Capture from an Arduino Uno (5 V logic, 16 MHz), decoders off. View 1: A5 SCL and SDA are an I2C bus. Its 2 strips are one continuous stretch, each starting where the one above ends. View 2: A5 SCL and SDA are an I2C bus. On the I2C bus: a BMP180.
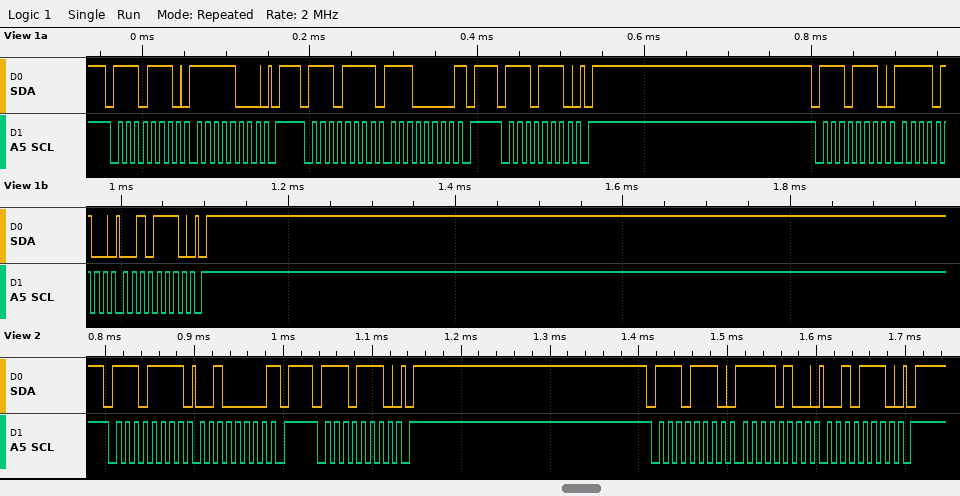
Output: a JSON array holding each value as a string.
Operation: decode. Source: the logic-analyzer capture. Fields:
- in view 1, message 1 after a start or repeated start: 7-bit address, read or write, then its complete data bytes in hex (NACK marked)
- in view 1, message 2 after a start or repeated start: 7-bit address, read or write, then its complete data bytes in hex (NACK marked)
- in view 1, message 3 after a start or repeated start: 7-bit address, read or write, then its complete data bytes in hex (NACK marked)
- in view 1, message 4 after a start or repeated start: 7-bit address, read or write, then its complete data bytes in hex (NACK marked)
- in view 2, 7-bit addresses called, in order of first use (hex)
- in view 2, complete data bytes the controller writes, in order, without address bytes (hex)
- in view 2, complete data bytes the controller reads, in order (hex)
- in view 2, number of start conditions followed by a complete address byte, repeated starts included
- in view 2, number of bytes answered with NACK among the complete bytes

["0x77 write: F8", "0x77 read: E0 NACK", "0x77 write", "0x77 write: F4 2E", "0x77", "F4 2E", "20", "3", "1"]
